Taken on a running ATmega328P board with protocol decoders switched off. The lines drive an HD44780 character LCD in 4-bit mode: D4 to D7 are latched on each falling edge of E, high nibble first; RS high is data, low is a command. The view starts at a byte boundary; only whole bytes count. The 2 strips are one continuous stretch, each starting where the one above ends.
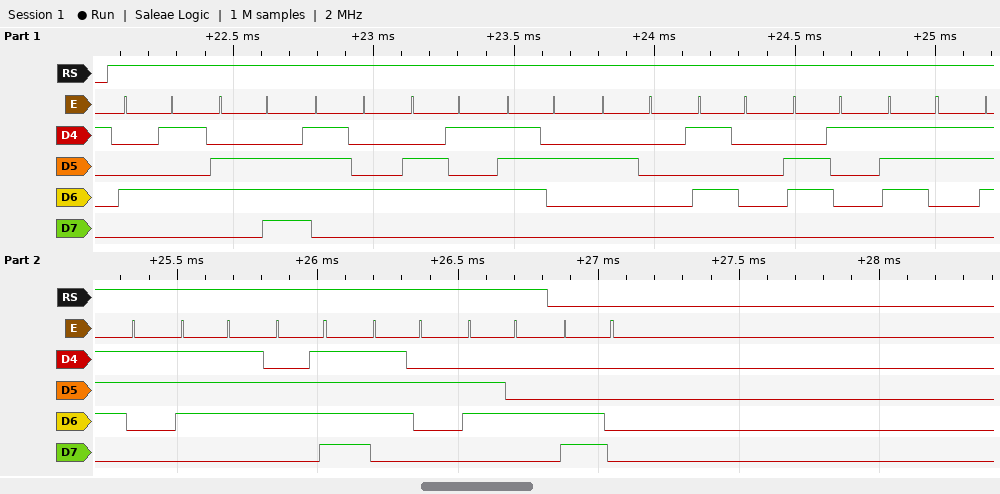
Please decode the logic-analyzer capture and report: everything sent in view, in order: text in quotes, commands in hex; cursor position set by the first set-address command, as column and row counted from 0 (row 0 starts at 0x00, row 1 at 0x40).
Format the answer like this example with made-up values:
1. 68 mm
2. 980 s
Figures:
1. "Enter Password" 0xC0
2. column 0, row 1
